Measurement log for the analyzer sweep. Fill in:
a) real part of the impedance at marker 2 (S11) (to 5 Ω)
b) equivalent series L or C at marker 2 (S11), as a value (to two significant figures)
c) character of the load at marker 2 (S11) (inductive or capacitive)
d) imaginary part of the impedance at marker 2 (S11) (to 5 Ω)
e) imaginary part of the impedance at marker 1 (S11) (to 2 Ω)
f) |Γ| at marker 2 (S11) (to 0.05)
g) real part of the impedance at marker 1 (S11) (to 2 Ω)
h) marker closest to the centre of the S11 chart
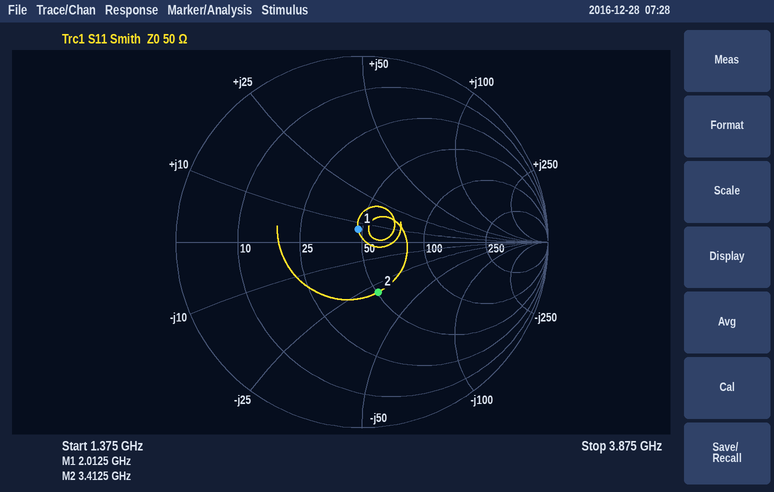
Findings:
50 Ω
1.6 pF
capacitive
-30 Ω
+6 Ω
0.30
48 Ω
marker 1
